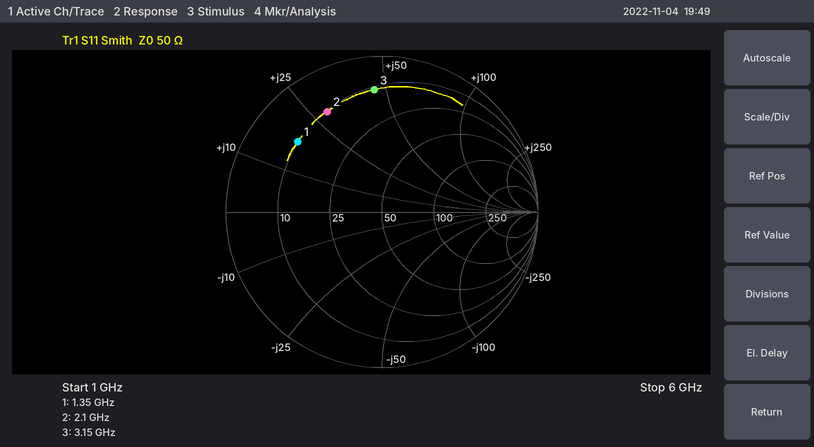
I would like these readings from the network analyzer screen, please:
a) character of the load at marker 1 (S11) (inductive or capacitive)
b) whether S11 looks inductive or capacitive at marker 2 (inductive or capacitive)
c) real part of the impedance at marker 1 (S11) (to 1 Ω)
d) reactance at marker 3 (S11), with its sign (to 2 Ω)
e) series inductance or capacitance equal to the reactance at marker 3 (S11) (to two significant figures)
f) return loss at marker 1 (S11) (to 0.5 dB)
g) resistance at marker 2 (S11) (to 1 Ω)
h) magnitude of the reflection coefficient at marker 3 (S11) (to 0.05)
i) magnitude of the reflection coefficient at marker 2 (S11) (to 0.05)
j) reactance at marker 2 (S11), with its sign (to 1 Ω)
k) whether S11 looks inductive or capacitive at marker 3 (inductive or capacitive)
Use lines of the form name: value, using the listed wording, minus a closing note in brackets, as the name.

character of the load at marker 1 (S11): inductive
whether S11 looks inductive or capacitive at marker 2: inductive
real part of the impedance at marker 1 (S11): 10 Ω
reactance at marker 3 (S11), with its sign: +46 Ω
series inductance or capacitance equal to the reactance at marker 3 (S11): 2.3 nH
return loss at marker 1 (S11): 3.0 dB
resistance at marker 2 (S11): 10 Ω
magnitude of the reflection coefficient at marker 3 (S11): 0.80
magnitude of the reflection coefficient at marker 2 (S11): 0.75
reactance at marker 2 (S11), with its sign: +29 Ω
whether S11 looks inductive or capacitive at marker 3: inductive
